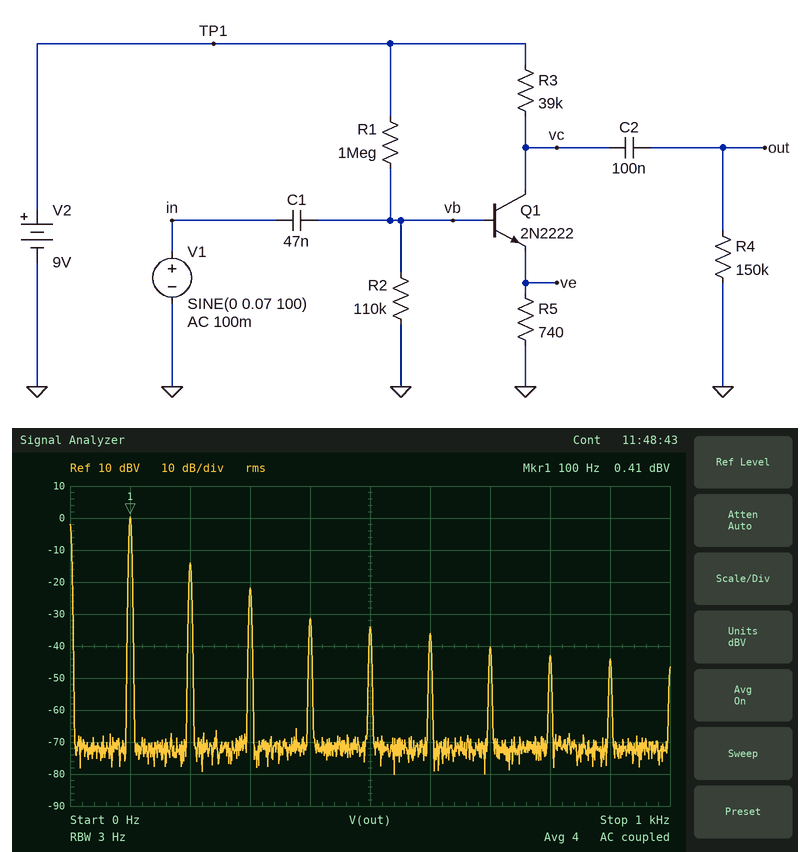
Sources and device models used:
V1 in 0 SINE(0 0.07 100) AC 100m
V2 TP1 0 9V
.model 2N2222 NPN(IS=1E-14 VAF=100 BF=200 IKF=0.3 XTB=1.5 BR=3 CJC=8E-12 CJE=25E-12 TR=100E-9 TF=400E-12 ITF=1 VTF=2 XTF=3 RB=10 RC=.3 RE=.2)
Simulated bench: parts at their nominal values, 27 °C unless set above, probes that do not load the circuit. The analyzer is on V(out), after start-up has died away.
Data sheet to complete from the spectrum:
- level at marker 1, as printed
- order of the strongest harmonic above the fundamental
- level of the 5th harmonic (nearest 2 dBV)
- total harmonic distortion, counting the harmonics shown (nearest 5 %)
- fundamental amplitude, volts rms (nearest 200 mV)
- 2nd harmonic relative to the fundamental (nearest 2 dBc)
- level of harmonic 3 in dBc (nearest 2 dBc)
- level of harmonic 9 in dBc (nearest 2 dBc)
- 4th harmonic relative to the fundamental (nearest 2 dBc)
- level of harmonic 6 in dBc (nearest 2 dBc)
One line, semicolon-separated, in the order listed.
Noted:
0.41 dBV; 2; -34 dBV; 20 %; 1.0 V; -14 dBc; -22 dBc; -44 dBc; -32 dBc; -36 dBc
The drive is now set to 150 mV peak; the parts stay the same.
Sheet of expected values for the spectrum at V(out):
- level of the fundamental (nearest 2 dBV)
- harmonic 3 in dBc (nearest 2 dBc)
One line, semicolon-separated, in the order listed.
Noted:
6 dBV; -20 dBc
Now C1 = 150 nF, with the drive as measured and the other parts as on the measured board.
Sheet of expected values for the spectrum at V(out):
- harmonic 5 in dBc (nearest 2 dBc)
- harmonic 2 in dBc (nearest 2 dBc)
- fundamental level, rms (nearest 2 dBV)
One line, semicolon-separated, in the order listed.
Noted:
-36 dBc; -22 dBc; 4 dBV
